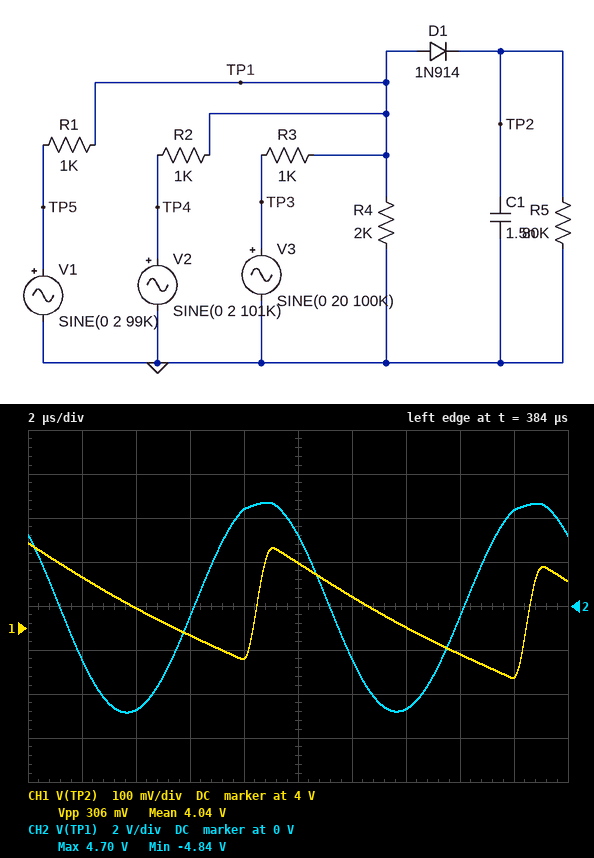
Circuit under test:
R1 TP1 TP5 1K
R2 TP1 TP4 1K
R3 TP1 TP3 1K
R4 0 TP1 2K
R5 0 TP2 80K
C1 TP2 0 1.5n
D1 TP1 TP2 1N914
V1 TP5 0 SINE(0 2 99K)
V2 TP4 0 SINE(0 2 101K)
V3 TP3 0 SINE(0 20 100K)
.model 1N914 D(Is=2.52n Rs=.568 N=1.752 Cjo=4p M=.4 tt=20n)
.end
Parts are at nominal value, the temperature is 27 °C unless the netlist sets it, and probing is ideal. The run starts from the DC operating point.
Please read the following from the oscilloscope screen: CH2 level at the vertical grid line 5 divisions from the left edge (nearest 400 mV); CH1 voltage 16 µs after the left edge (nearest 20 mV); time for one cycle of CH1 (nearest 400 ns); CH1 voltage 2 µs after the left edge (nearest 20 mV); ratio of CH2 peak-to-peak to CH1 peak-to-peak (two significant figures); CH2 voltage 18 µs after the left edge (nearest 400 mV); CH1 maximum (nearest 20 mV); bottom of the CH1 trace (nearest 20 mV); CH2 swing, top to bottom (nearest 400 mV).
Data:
3.2 V
3.94 V
10.0 µs
4.12 V
31
4.4 V
4.20 V
3.88 V
9.6 V
